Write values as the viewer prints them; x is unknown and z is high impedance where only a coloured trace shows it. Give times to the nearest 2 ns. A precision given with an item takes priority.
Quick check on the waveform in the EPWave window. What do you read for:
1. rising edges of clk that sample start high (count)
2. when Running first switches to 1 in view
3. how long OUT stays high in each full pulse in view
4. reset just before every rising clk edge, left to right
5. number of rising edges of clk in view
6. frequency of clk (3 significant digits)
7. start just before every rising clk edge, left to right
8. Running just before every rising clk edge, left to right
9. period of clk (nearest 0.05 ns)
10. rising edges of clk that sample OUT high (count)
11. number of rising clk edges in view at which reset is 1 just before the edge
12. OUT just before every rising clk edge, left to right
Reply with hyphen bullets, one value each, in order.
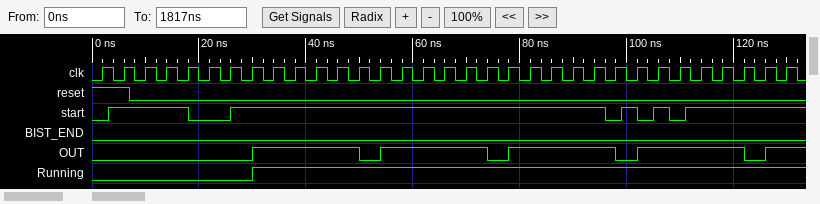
- 28
- 30 ns
- 20 ns, 20 ns, 20 ns, 20 ns
- 1 1 0 0 0 0 0 0 0 0 0 0 0 0 0 0 0 0 0 0 0 0 0 0 0 0 0 0 0 0 0 0 0
- 33
- 250 MHz
- 0 1 1 1 1 0 0 1 1 1 1 1 1 1 1 1 1 1 1 1 1 1 1 1 0 1 1 0 1 1 1 1 1
- 0 0 0 0 0 0 0 0 1 1 1 1 1 1 1 1 1 1 1 1 1 1 1 1 1 1 1 1 1 1 1 1 1
- 4 ns
- 21
- 2
- 0 0 0 0 0 0 0 0 1 1 1 1 1 0 1 1 1 1 1 0 1 1 1 1 1 0 1 1 1 1 1 0 1
